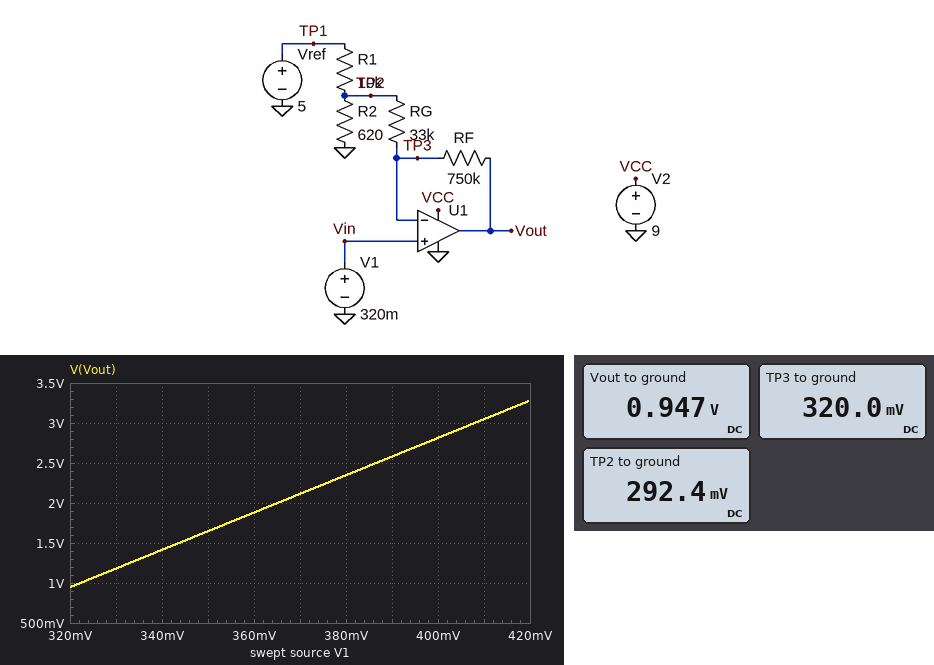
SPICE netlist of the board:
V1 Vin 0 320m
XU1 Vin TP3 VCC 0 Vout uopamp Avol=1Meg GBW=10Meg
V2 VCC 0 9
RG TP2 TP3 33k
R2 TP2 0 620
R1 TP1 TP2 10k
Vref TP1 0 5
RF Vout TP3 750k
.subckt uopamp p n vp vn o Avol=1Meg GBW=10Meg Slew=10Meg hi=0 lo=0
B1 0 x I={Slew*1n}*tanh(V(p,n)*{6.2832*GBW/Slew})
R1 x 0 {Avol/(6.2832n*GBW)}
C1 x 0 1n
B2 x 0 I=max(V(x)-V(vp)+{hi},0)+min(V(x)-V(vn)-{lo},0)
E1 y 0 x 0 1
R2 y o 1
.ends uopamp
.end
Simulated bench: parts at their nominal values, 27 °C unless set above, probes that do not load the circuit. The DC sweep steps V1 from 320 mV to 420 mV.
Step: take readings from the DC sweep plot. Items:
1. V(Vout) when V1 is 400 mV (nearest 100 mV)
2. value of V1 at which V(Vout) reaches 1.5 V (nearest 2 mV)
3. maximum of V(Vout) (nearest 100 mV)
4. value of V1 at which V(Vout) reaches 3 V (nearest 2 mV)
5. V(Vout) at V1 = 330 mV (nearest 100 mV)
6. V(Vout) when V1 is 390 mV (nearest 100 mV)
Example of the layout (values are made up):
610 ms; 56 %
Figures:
2.8 V; 344 mV; 3.3 V; 408 mV; 1.2 V; 2.6 V
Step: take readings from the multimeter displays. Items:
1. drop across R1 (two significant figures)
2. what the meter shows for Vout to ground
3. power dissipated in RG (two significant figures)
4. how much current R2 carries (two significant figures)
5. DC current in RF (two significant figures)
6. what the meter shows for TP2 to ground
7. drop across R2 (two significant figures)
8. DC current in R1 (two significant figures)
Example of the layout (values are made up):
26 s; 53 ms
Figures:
4.7 V; 0.947 V; 23 nW; 470 µA; 840 nA; 292.4 mV; 290 mV; 470 µA
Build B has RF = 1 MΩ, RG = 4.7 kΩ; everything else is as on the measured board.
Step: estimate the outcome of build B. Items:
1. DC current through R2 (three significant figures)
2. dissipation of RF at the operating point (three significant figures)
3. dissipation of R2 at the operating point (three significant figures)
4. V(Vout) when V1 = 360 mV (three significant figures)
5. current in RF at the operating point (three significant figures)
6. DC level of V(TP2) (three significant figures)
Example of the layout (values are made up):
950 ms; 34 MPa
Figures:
476 µA; 28.3 µW; 140 µW; 9.00 V; 5.32 µA; 295 mV
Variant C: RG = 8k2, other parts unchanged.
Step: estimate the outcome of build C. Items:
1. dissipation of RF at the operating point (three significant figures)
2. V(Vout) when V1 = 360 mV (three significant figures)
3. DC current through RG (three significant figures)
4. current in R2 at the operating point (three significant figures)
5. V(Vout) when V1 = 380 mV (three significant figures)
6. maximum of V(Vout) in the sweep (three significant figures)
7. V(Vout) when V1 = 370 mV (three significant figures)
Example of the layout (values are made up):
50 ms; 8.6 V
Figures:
7.67 µW; 6.17 V; 3.20 µA; 474 µA; 7.90 V; 9.00 V; 7.04 V
